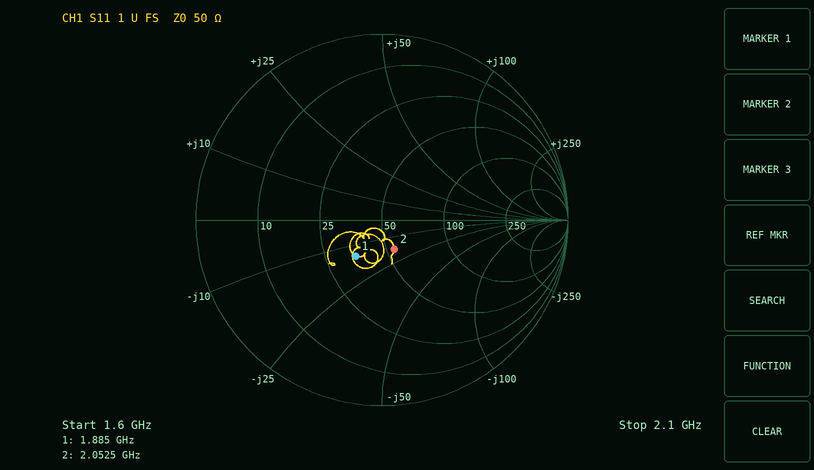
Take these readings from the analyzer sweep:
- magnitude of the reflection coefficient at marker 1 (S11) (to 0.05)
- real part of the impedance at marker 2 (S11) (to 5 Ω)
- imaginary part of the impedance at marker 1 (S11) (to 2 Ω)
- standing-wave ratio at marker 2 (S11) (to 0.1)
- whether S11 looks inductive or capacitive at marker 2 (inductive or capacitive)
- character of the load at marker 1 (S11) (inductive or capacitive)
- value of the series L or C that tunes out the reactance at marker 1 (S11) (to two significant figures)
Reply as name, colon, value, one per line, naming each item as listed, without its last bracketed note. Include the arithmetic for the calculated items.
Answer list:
magnitude of the reflection coefficient at marker 1 (S11): 0.25
real part of the impedance at marker 2 (S11): 55 Ω
imaginary part of the impedance at marker 1 (S11): -14 Ω
standing-wave ratio at marker 2 (S11): 1.4
whether S11 looks inductive or capacitive at marker 2: capacitive
character of the load at marker 1 (S11): capacitive
value of the series L or C that tunes out the reactance at marker 1 (S11): L = 14 Ω/(2π × 1.885 GHz) ≈ 1.2 nH
